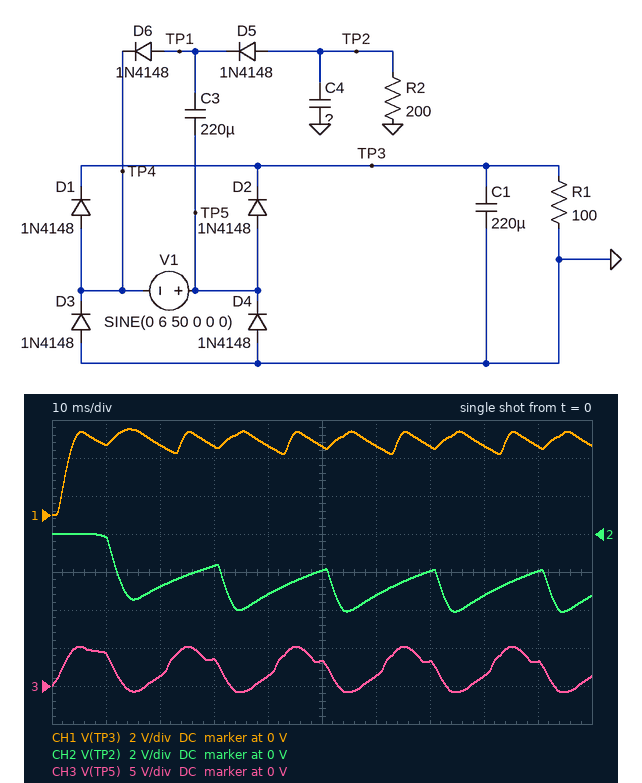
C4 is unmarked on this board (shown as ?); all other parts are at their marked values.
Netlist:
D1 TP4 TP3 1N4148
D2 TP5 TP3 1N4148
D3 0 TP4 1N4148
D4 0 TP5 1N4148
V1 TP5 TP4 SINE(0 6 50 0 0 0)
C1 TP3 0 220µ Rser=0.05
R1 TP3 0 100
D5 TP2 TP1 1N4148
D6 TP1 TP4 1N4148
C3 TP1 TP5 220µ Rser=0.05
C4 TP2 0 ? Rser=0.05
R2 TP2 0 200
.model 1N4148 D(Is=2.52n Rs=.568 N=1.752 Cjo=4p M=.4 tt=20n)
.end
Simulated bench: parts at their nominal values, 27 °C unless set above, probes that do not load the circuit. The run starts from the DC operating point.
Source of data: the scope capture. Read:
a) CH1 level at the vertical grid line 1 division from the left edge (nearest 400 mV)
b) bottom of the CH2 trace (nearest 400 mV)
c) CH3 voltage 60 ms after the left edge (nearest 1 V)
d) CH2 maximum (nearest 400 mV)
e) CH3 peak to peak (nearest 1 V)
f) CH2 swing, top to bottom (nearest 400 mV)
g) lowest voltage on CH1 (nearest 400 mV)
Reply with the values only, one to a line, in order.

3.6 V
-4.0 V
1 V
0 V
6 V
4.0 V
0 V
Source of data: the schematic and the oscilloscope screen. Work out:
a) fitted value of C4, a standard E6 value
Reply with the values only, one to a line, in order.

100 µF
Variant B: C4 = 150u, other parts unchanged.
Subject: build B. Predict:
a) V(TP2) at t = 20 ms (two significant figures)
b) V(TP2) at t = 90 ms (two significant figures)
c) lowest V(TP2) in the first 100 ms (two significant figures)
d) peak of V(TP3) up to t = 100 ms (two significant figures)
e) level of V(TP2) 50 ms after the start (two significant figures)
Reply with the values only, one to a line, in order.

-2.5 V
-2.4 V
-4.0 V
4.8 V
-2.3 V
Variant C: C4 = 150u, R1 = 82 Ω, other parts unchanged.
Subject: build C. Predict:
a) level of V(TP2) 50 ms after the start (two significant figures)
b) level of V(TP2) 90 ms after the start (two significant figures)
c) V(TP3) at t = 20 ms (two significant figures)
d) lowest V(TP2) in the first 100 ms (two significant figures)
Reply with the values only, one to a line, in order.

-2.3 V
-2.4 V
3.5 V
-4.0 V
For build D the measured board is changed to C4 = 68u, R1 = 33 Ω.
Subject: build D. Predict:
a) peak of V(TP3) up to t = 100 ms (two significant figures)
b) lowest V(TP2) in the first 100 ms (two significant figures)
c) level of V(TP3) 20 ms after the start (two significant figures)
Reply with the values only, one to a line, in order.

4.2 V
-4.4 V
2.4 V
